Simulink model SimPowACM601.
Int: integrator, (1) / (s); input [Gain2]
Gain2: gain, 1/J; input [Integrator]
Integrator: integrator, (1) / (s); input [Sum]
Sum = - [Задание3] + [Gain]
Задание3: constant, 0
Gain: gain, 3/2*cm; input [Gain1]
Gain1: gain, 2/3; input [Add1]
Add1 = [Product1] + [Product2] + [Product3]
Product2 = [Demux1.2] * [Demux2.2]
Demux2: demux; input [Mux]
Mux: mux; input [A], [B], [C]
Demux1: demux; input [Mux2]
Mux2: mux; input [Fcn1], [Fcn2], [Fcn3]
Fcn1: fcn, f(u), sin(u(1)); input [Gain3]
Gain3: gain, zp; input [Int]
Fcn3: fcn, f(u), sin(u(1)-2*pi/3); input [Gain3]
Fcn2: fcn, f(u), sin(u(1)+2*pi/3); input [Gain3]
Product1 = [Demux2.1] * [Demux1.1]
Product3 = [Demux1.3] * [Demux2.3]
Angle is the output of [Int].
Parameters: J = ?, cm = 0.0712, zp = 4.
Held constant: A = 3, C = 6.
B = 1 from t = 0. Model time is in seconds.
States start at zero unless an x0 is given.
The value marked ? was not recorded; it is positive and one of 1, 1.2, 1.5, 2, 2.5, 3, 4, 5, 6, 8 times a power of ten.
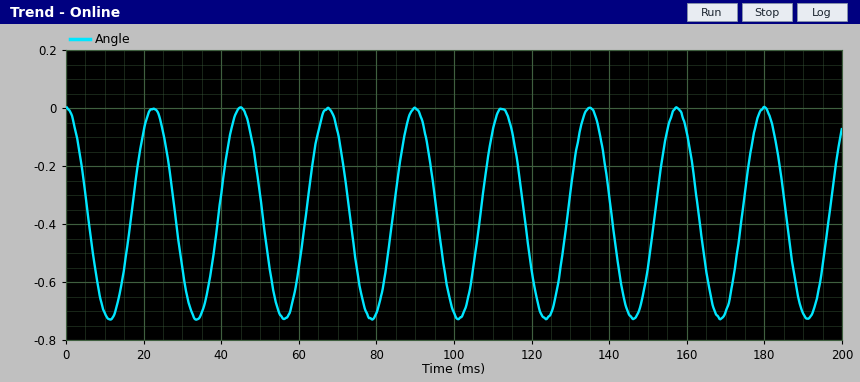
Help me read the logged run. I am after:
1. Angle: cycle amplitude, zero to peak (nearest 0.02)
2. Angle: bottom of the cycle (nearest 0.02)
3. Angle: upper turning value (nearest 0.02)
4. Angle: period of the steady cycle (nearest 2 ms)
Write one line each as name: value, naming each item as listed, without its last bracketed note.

Angle: cycle amplitude, zero to peak: 0.36
Angle: bottom of the cycle: -0.72
Angle: upper turning value: 0.00
Angle: period of the steady cycle: 22 ms
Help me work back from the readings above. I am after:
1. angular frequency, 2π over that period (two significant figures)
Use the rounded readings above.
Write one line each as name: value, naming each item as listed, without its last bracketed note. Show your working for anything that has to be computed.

angular frequency, 2π over that period: 2π / 22 = 0.29 rad/ms
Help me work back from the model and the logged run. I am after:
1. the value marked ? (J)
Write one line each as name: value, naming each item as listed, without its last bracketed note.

the value marked ?: 1.2e-05
